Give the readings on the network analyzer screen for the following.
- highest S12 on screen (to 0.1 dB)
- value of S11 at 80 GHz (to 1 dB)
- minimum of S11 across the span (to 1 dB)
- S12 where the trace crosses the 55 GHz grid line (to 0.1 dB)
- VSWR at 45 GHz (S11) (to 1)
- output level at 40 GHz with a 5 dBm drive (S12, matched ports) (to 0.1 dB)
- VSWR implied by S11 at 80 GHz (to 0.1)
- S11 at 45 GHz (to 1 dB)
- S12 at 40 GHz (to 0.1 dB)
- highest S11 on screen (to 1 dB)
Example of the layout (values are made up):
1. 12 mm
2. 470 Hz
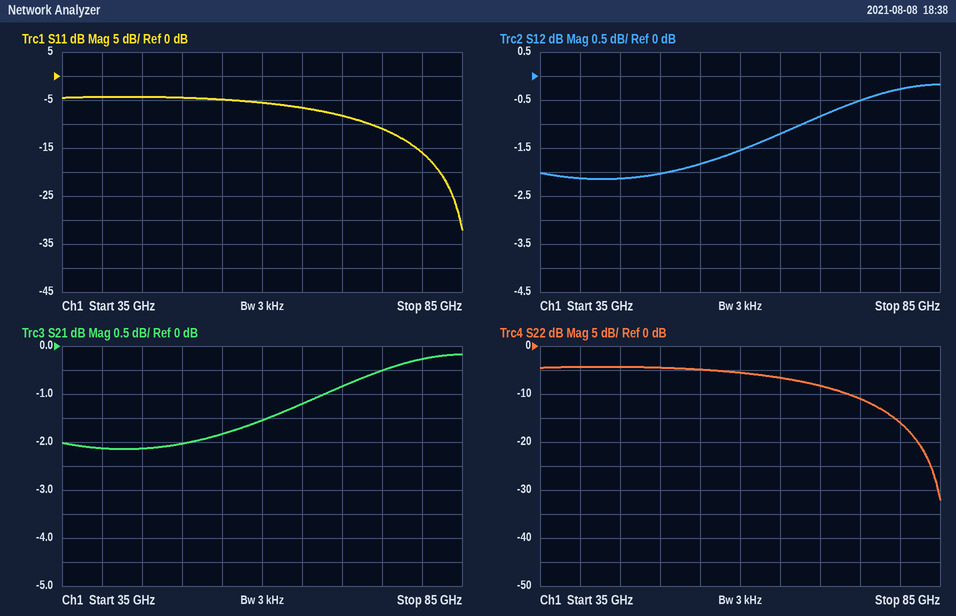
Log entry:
1. -0.2 dB
2. -16 dB
3. -32 dB
4. -1.8 dB
5. 4
6. 2.9 dBm
7. 1.4
8. -4 dB
9. -2.1 dB
10. -4 dB
